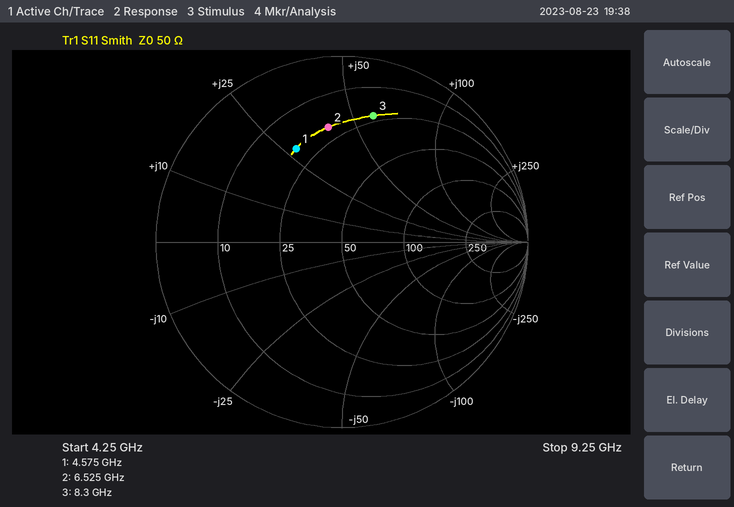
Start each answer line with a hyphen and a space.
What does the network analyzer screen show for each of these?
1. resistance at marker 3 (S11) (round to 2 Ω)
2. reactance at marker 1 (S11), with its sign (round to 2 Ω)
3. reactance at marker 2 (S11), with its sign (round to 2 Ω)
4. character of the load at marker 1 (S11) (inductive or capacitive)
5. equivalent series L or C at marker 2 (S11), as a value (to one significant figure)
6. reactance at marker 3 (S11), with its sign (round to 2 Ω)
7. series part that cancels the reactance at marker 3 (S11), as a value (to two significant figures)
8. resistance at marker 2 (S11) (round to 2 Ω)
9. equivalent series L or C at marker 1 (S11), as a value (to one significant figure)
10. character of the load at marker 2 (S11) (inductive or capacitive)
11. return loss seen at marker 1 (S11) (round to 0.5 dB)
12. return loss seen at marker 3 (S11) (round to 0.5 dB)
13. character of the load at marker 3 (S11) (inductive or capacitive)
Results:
- 22 Ω
- +28 Ω
- +40 Ω
- inductive
- 1.0 nH
- +58 Ω
- 330 fF
- 20 Ω
- 1.0 nH
- inductive
- 5.0 dB
- 3.0 dB
- inductive
